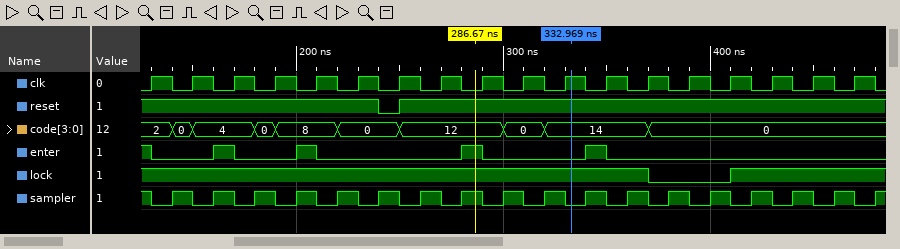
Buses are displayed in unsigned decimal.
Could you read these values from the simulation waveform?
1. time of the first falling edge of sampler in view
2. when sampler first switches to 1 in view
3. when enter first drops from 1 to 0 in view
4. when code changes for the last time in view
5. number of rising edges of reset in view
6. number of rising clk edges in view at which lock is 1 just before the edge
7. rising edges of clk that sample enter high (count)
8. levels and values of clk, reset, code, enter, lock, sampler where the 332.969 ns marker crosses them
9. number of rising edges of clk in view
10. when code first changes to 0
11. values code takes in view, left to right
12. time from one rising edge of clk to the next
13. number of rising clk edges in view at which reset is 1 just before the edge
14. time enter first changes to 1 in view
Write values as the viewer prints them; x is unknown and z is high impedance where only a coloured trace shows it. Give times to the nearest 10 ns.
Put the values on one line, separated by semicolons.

130 ns; 140 ns; 130 ns; 370 ns; 1; 16; 5; clk=1, reset=1, code=14, enter=0, lock=1, sampler=0; 18; 140 ns; 2, 0, 4, 0, 8, 0, 12, 0, 14, 0; 20 ns; 17; 160 ns
